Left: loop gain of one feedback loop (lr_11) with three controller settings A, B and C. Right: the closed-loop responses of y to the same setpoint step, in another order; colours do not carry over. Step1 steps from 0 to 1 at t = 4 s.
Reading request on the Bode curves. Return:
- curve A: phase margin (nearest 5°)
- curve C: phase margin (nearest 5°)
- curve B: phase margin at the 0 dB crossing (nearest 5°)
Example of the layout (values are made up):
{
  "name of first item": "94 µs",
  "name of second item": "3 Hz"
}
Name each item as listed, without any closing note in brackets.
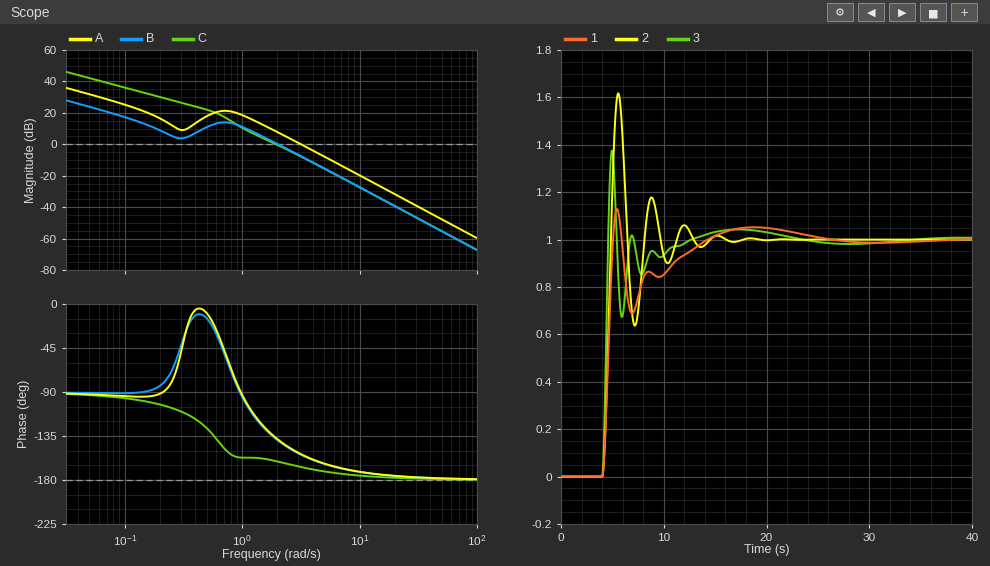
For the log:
{
  "curve A: phase margin": "25°",
  "curve C: phase margin": "20°",
  "curve B: phase margin at the 0 dB crossing": "40°"
}
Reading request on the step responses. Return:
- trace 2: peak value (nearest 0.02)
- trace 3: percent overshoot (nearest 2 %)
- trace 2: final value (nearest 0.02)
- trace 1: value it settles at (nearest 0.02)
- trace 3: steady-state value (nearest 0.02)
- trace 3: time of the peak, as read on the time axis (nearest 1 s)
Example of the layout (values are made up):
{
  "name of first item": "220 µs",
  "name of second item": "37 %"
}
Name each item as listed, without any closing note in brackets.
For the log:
{
  "trace 2: peak value": "1.62",
  "trace 3: percent overshoot": "38 %",
  "trace 2: final value": "1.00",
  "trace 1: value it settles at": "1.00",
  "trace 3: steady-state value": "1.00",
  "trace 3: time of the peak, as read on the time axis": "5 s"
}
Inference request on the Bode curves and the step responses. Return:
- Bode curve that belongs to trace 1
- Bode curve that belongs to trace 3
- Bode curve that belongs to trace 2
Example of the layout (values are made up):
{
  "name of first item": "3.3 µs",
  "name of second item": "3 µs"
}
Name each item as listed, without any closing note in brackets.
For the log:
{
  "Bode curve that belongs to trace 1": "B",
  "Bode curve that belongs to trace 3": "A",
  "Bode curve that belongs to trace 2": "C"
}
